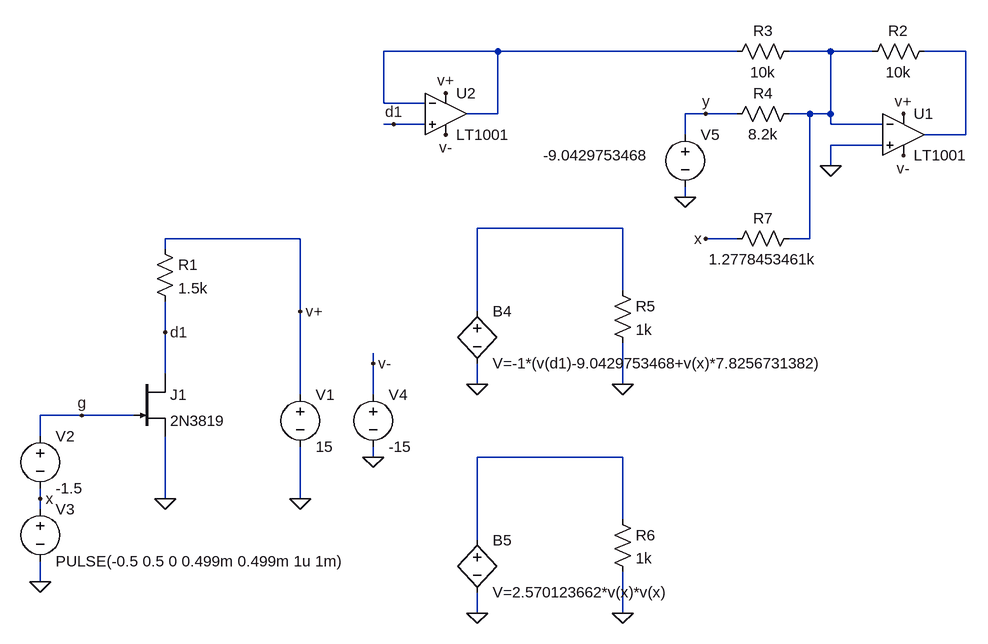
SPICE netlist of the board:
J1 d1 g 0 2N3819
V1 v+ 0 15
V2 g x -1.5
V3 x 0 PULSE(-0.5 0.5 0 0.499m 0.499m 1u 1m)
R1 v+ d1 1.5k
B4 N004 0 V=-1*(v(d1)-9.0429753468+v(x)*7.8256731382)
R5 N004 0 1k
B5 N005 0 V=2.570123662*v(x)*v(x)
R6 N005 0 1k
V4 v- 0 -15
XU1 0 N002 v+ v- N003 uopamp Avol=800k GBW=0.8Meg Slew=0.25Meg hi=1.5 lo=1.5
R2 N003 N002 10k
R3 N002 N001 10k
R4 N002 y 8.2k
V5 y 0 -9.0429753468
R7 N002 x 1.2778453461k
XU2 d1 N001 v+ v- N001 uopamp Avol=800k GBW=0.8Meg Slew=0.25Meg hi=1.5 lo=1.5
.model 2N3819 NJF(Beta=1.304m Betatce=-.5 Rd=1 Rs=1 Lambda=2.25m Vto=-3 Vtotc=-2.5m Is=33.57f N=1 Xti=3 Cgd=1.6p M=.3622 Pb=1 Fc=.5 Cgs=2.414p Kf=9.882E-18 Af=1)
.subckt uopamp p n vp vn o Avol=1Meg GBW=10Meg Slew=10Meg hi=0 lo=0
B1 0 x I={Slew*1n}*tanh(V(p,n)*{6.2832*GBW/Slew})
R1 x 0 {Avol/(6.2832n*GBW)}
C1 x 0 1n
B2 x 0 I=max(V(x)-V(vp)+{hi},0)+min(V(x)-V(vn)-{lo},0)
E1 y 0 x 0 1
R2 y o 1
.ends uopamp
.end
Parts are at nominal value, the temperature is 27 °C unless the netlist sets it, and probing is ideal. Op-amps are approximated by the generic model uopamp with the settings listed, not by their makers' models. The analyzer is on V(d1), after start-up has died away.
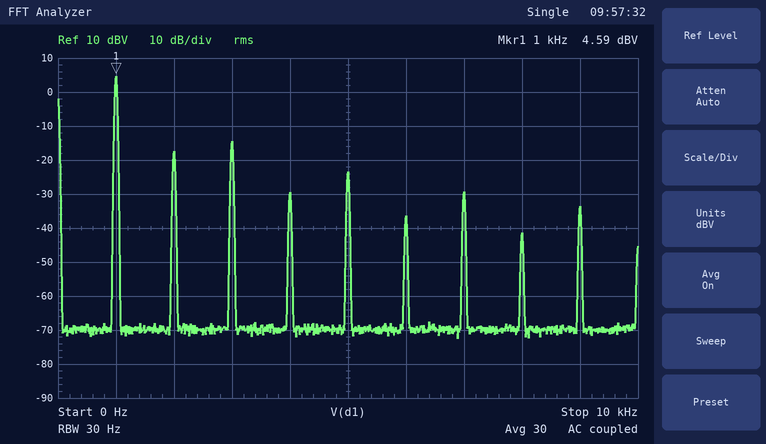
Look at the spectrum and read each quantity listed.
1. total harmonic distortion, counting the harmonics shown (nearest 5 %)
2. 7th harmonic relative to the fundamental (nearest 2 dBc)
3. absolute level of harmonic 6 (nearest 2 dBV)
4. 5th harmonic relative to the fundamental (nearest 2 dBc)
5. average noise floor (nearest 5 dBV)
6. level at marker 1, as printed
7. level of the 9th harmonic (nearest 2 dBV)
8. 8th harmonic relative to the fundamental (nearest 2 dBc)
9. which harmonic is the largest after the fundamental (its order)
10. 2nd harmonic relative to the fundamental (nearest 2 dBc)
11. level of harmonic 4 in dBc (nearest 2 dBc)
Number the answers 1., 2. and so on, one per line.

1. 15 %
2. -34 dBc
3. -36 dBV
4. -28 dBc
5. -70 dBV
6. 4.59 dBV
7. -34 dBV
8. -46 dBc
9. 3
10. -22 dBc
11. -34 dBc
